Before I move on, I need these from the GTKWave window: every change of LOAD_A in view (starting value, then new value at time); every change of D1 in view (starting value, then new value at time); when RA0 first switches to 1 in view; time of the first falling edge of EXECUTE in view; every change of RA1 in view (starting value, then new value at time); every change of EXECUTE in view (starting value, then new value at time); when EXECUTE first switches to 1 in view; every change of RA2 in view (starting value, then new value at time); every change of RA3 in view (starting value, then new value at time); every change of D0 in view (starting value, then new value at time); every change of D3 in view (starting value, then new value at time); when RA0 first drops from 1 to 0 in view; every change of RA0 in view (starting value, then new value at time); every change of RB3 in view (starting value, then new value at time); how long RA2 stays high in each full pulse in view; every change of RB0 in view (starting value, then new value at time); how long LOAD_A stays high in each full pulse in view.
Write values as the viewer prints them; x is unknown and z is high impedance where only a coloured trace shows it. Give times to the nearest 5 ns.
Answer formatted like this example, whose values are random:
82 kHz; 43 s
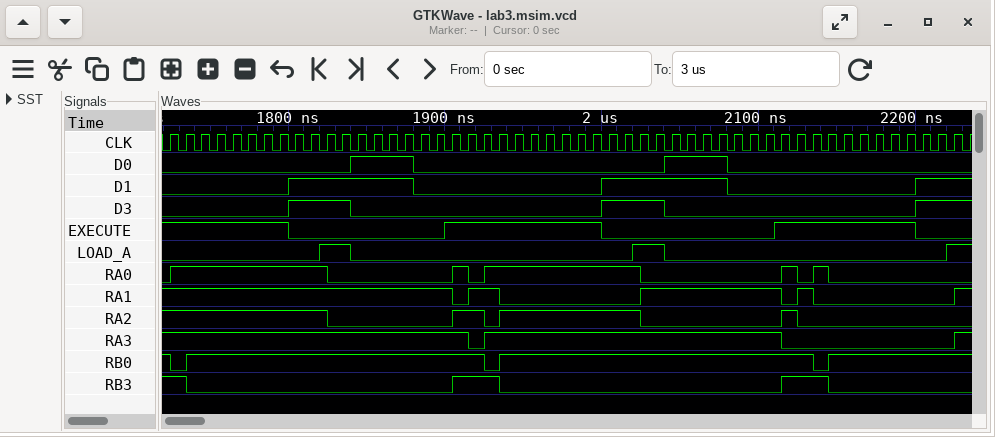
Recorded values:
0, 1 at 1820 ns, 0 at 1840 ns, 1 at 2020 ns, 0 at 2040 ns, 1 at 2220 ns; 0, 1 at 1800 ns, 0 at 1880 ns, 1 at 2000 ns, 0 at 2080 ns, 1 at 2200 ns; 1725 ns; 1800 ns; 1, 0 at 1905 ns, 1 at 1915 ns, 0 at 1935 ns, 1 at 2025 ns, 0 at 2115 ns, 1 at 2125 ns, 0 at 2135 ns, 1 at 2225 ns; 1, 0 at 1800 ns, 1 at 1900 ns, 0 at 2000 ns, 1 at 2110 ns, 0 at 2200 ns; 1900 ns; 1, 0 at 1825 ns, 1 at 1905 ns, 0 at 1925 ns, 1 at 1935 ns, 0 at 2025 ns, 1 at 2115 ns, 0 at 2125 ns; 1, 0 at 1915 ns, 1 at 1925 ns, 0 at 2115 ns, 1 at 2225 ns; 0, 1 at 1840 ns, 0 at 1880 ns, 1 at 2040 ns, 0 at 2080 ns; 0, 1 at 1800 ns, 0 at 1840 ns, 1 at 2000 ns, 0 at 2040 ns, 1 at 2200 ns; 1825 ns; 0, 1 at 1725 ns, 0 at 1825 ns, 1 at 1905 ns, 0 at 1915 ns, 1 at 1925 ns, 0 at 2025 ns, 1 at 2115 ns, 0 at 2125 ns, 1 at 2135 ns, 0 at 2145 ns; 1, 0 at 1735 ns, 1 at 1905 ns, 0 at 1935 ns, 1 at 2115 ns, 0 at 2145 ns; 20 ns, 90 ns, 10 ns; 1, 0 at 1725 ns, 1 at 1735 ns, 0 at 1925 ns, 1 at 1935 ns, 0 at 2135 ns, 1 at 2145 ns; 20 ns, 20 ns
